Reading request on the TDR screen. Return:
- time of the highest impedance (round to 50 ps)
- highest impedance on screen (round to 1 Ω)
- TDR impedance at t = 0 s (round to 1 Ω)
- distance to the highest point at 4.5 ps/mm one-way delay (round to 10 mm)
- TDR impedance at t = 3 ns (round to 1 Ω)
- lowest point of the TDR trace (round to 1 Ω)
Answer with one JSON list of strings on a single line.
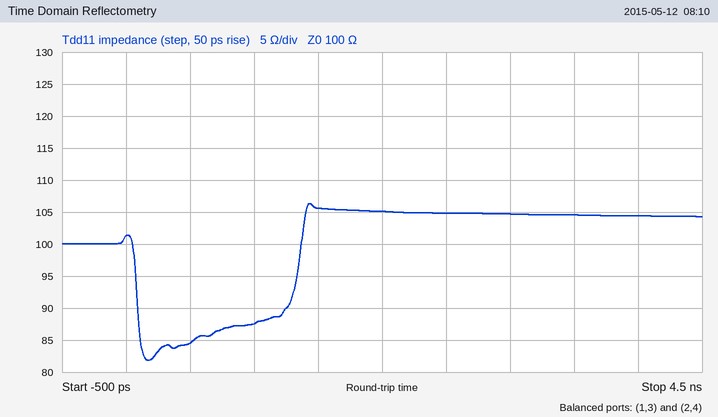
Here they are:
["1.45 ns", "106 Ω", "101 Ω", "160 mm", "105 Ω", "82 Ω"]
